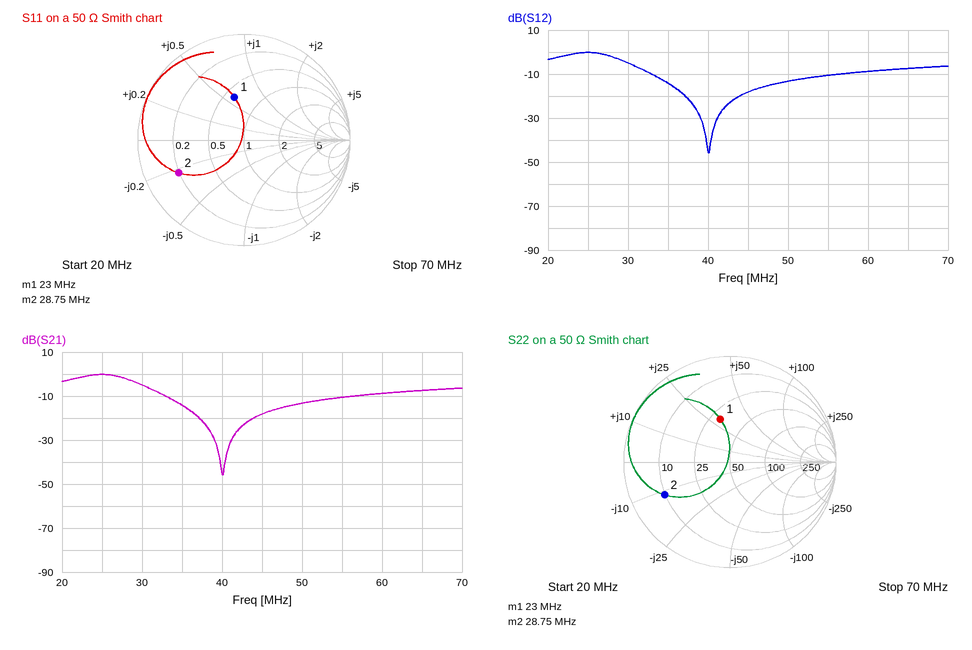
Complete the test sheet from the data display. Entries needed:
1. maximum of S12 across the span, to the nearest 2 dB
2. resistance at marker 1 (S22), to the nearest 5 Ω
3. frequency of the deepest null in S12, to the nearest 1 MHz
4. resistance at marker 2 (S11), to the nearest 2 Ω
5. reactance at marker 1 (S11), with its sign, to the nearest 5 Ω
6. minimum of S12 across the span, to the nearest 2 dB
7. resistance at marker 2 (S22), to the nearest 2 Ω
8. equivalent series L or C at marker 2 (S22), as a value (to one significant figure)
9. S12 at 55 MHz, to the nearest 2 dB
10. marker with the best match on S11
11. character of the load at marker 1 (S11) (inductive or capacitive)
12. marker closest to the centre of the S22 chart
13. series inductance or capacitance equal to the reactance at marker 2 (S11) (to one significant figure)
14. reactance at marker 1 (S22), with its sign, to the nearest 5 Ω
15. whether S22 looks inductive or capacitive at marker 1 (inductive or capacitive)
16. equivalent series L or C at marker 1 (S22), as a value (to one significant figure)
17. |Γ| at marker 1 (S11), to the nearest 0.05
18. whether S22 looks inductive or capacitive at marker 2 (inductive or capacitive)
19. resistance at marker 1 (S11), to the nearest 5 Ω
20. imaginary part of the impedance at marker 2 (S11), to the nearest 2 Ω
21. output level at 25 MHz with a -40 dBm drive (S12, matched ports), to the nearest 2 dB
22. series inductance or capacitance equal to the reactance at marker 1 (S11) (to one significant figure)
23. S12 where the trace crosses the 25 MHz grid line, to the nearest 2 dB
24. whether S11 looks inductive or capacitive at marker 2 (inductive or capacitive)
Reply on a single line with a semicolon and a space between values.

0 dB; 30 Ω; 40 MHz; 10 Ω; +30 Ω; -46 dB; 10 Ω; 500 pF; -10 dB; marker 1; inductive; marker 1; 500 pF; +30 Ω; inductive; 200 nH; 0.40; capacitive; 30 Ω; -12 Ω; -40 dBm; 200 nH; 0 dB; capacitive
